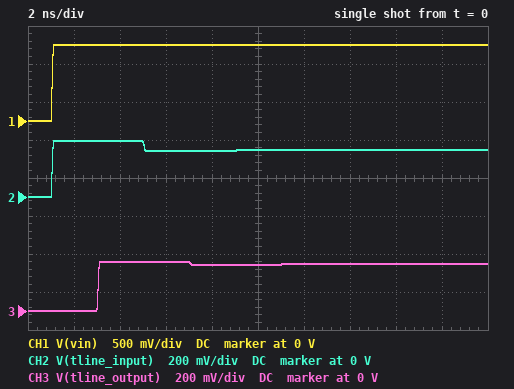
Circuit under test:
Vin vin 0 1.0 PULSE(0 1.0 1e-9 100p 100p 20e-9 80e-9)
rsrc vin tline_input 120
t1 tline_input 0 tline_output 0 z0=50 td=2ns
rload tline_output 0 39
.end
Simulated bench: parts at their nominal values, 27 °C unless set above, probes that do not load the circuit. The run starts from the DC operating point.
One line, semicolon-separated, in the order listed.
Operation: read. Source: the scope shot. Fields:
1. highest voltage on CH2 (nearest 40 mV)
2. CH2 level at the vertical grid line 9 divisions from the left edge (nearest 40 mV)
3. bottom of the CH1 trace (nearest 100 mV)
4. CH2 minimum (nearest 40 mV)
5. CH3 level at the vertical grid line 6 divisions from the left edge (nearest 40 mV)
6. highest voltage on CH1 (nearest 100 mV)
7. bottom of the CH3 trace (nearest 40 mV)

280 mV; 240 mV; 0 V; 0 V; 240 mV; 1.0 V; 0 V
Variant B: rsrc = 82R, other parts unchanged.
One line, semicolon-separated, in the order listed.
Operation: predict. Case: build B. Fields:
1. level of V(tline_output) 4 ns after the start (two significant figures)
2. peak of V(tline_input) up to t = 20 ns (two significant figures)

330 mV; 380 mV
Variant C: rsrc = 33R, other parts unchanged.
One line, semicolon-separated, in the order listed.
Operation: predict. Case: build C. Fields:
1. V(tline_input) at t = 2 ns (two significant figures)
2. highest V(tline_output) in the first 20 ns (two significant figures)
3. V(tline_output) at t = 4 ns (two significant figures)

600 mV; 540 mV; 530 mV
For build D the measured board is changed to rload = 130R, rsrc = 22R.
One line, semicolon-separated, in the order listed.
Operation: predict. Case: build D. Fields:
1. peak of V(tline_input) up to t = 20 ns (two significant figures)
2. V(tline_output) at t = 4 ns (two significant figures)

880 mV; 1.0 V
